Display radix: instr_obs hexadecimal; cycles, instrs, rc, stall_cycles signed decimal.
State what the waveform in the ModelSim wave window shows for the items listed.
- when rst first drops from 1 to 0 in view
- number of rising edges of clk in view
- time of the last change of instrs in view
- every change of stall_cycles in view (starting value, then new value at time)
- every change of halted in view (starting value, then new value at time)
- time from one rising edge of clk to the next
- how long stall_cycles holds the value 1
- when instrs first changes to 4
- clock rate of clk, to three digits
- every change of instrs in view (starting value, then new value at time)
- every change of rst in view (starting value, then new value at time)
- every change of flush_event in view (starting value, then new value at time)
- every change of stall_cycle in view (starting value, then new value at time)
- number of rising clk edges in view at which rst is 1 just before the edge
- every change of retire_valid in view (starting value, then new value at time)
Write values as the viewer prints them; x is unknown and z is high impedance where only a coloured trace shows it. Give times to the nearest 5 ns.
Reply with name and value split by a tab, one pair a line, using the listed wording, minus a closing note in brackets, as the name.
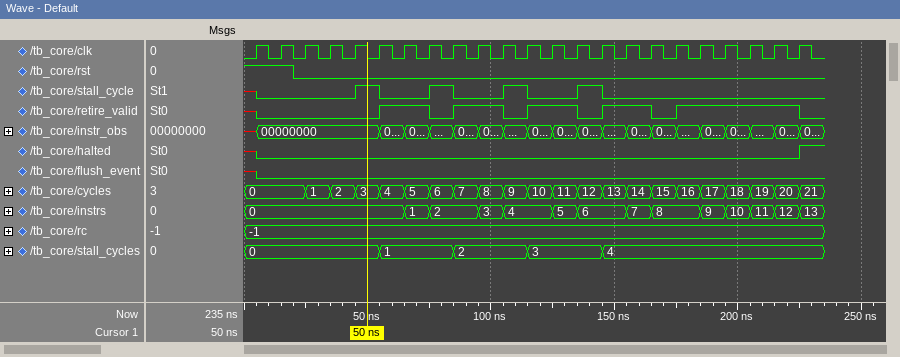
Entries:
when rst first drops from 1 to 0 in view	20 ns
number of rising edges of clk in view	23
time of the last change of instrs in view	225 ns
every change of stall_cycles in view	0, 1 at 55 ns, 2 at 85 ns, 3 at 115 ns, 4 at 145 ns
every change of halted in view	x, 0 at 5 ns, 1 at 225 ns
time from one rising edge of clk to the next	10 ns
how long stall_cycles holds the value 1	30 ns
when instrs first changes to 4	105 ns
clock rate of clk, to three digits	100 MHz
every change of instrs in view	0, 1 at 65 ns, 2 at 75 ns, 3 at 95 ns, 4 at 105 ns, 5 at 125 ns, 6 at 135 ns, 7 at 155 ns, 8 at 165 ns, 9 at 185 ns, 10 at 195 ns, 11 at 205 ns, 12 at 215 ns, 13 at 225 ns
every change of rst in view	1, 0 at 20 ns
every change of flush_event in view	x, 0 at 5 ns
every change of stall_cycle in view	x, 0 at 5 ns, 1 at 45 ns, 0 at 55 ns, 1 at 75 ns, 0 at 85 ns, 1 at 105 ns, 0 at 115 ns, 1 at 135 ns, 0 at 145 ns
number of rising clk edges in view at which rst is 1 just before the edge	2
every change of retire_valid in view	x, 0 at 5 ns, 1 at 55 ns, 0 at 75 ns, 1 at 85 ns, 0 at 105 ns, 1 at 115 ns, 0 at 135 ns, 1 at 145 ns, 0 at 165 ns, 1 at 175 ns, 0 at 225 ns
